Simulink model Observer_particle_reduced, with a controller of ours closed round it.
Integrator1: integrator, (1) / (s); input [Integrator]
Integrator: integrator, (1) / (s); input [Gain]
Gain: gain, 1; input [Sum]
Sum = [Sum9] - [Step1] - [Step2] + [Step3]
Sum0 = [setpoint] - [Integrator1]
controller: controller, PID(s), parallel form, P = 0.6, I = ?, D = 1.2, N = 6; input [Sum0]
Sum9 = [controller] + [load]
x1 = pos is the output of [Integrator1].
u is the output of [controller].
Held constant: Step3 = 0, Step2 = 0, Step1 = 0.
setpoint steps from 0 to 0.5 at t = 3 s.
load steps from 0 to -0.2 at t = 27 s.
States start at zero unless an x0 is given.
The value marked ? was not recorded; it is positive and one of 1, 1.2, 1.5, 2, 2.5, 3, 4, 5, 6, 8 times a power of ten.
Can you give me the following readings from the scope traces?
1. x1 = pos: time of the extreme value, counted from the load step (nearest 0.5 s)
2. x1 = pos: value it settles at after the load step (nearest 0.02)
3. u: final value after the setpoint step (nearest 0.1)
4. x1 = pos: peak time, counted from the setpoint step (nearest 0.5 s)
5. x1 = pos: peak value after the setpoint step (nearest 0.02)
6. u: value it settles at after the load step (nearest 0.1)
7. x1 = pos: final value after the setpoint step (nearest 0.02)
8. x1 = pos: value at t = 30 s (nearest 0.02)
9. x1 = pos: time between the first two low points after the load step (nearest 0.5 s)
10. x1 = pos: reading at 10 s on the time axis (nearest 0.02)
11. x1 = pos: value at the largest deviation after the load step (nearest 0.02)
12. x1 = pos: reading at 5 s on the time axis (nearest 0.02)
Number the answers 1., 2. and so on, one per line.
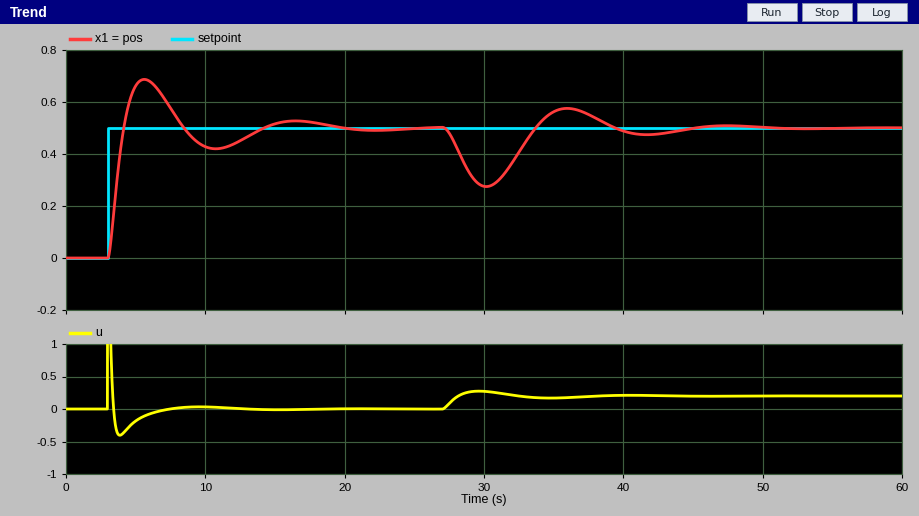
1. 3.0 s
2. 0.50
3. 0.0
4. 2.5 s
5. 0.68
6. 0.2
7. 0.50
8. 0.28
9. 11.5 s
10. 0.42
11. 0.28
12. 0.66
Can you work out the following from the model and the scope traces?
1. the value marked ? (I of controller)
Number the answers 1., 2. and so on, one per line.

1. 0.3
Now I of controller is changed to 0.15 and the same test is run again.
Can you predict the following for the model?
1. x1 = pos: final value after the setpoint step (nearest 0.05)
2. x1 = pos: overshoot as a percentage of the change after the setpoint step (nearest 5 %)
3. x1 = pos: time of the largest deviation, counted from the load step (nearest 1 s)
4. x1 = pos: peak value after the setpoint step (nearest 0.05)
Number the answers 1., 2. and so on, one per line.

1. 0.50
2. 30 %
3. 4 s
4. 0.65
